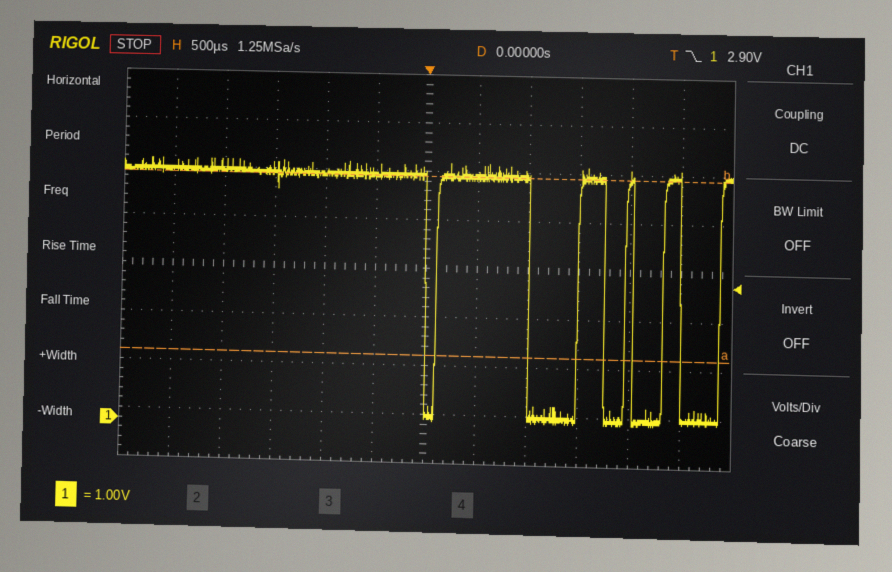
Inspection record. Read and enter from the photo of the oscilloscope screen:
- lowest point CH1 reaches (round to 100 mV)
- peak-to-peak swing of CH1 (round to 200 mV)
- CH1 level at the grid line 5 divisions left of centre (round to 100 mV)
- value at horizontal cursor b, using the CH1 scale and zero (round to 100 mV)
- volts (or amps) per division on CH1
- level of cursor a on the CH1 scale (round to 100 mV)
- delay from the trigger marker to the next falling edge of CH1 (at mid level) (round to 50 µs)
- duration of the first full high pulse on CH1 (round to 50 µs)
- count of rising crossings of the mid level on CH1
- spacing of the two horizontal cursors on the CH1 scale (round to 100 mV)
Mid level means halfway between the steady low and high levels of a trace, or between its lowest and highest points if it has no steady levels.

100 mV
5.2 V
5.2 V
5.1 V
1 V
1.4 V
1.00 ms
900 µs
5
3.7 V
